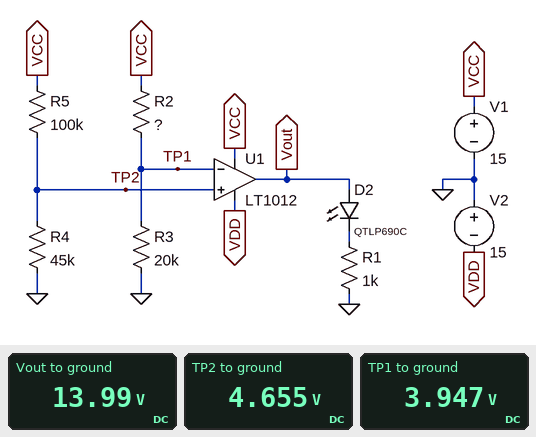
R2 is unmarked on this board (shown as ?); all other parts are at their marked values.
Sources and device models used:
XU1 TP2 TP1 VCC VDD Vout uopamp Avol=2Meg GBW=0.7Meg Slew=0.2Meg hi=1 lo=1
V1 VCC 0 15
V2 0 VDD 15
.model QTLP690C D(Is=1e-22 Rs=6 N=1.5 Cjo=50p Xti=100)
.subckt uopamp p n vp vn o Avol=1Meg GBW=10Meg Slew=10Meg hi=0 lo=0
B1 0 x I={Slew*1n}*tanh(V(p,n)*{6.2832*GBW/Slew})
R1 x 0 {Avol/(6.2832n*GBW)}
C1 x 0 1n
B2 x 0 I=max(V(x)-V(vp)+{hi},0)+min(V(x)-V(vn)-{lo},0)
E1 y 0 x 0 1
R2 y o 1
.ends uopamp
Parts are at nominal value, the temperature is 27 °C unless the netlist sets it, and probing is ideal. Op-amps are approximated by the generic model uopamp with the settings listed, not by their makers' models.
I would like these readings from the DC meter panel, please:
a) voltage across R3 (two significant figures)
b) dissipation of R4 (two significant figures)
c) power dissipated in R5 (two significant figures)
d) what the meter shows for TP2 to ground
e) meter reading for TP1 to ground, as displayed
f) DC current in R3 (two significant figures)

3.9 V
480 µW
1.1 mW
4.655 V
3.947 V
200 µA
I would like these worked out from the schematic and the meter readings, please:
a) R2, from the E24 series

56 kΩ
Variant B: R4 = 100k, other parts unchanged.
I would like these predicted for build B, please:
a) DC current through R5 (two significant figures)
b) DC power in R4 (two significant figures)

75 µA
560 µW
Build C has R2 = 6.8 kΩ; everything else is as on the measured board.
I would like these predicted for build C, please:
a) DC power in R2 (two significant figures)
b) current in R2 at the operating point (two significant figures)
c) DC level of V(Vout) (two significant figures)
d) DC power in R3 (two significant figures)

2.1 mW
560 µA
-14 V
6.3 mW
